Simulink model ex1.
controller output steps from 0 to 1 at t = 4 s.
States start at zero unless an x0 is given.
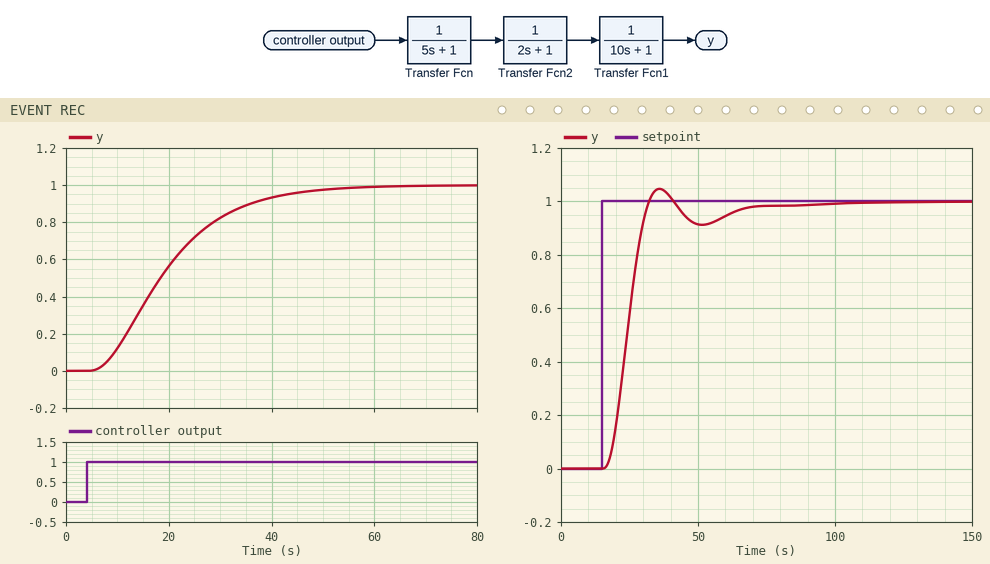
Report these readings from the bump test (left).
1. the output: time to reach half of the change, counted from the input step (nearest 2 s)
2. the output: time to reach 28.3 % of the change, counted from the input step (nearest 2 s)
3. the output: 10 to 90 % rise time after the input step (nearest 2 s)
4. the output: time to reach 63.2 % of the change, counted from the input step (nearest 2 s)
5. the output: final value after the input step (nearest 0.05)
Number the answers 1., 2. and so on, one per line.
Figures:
1. 14 s
2. 10 s
3. 26 s
4. 18 s
5. 1.00
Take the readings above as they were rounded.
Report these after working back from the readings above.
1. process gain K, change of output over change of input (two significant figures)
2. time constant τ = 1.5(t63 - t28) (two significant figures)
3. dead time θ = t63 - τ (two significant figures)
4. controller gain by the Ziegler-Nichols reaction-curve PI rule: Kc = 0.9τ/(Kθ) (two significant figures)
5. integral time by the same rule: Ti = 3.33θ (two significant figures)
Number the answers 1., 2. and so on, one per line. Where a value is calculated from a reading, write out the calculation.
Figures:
1. (1 - 0) / 1 = 1.0
2. 1.5 × (18 - 10) = 12 s
3. 18 - 12 = 6.0 s
4. 0.9 × 12 / (1 × 6) = 1.8
5. 3.33 × 6 = 20 s
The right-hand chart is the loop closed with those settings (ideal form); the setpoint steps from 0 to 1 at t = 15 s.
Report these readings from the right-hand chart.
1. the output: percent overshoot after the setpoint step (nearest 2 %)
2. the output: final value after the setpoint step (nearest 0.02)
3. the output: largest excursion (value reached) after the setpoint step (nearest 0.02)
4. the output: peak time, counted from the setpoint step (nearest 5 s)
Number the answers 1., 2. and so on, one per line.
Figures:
1. 4 %
2. 1.00
3. 1.04
4. 20 s
